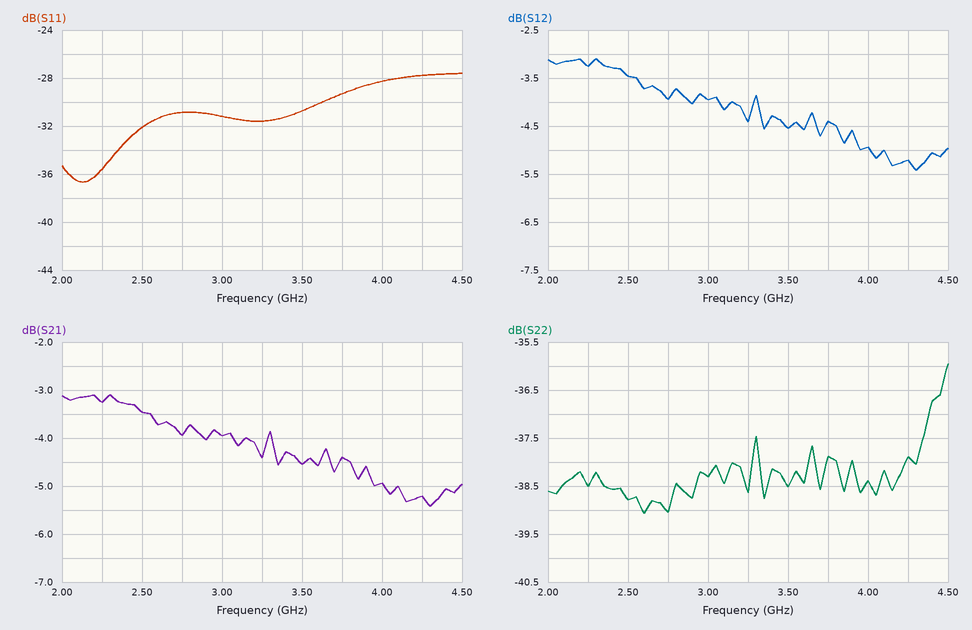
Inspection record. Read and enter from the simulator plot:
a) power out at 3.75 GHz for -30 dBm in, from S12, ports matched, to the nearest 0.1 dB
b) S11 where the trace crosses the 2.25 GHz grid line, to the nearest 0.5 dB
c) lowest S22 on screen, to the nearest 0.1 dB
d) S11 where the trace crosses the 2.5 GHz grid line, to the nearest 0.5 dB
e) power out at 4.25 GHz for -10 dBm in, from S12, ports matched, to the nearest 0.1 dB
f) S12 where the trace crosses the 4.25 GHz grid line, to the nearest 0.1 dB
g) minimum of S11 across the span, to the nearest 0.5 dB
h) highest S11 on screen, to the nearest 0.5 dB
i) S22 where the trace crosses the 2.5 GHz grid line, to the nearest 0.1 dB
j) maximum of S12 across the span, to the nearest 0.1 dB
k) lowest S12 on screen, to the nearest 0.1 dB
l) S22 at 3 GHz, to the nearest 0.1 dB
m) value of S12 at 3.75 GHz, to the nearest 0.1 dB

-34.4 dBm
-35.5 dB
-39.1 dB
-32.0 dB
-15.2 dBm
-5.2 dB
-36.5 dB
-27.5 dB
-38.8 dB
-3.1 dB
-5.4 dB
-38.3 dB
-4.4 dB
